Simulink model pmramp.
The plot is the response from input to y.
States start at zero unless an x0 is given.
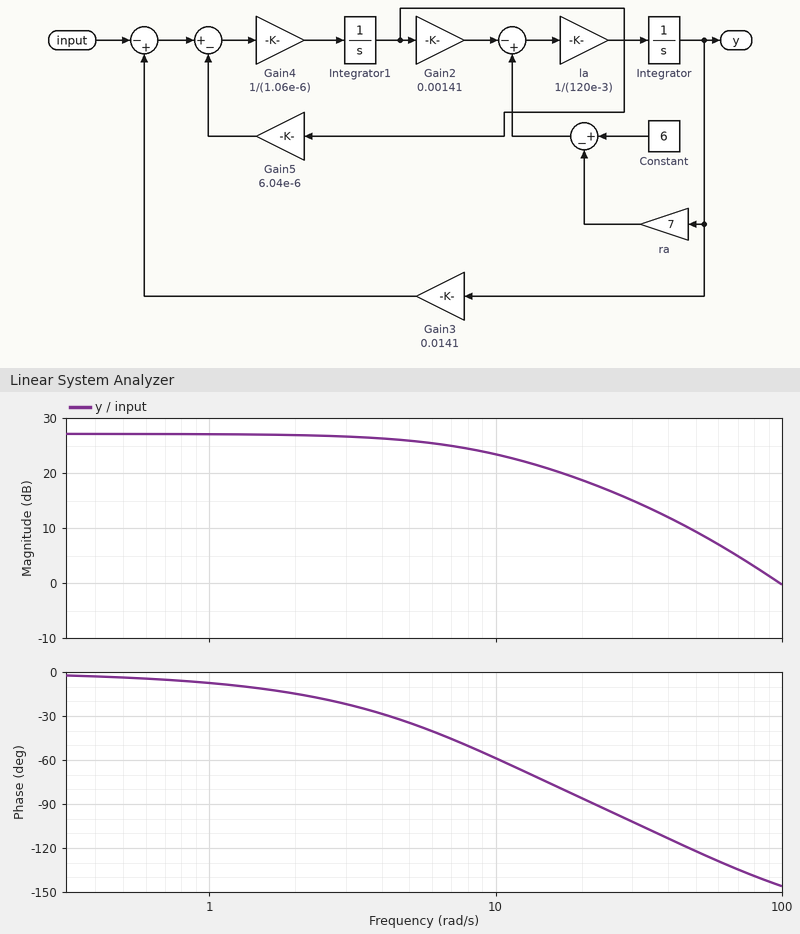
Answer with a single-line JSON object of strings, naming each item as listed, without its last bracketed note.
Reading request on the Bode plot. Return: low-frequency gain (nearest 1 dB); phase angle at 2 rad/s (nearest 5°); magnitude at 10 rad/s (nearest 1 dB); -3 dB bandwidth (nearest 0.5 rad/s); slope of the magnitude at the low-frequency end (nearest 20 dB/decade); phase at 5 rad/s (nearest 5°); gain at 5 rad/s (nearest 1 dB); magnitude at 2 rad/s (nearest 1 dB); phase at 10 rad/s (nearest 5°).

{"low-frequency gain": "27 dB", "phase angle at 2 rad/s": "-15°", "magnitude at 10 rad/s": "23 dB", "-3 dB bandwidth": "8.5 rad/s", "slope of the magnitude at the low-frequency end": "0 dB/decade", "phase at 5 rad/s": "-35°", "gain at 5 rad/s": "26 dB", "magnitude at 2 rad/s": "27 dB", "phase at 10 rad/s": "-60°"}
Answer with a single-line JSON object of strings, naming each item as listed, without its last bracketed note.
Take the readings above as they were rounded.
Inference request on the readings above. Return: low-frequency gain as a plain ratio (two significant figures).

{"low-frequency gain as a plain ratio": "22"}
